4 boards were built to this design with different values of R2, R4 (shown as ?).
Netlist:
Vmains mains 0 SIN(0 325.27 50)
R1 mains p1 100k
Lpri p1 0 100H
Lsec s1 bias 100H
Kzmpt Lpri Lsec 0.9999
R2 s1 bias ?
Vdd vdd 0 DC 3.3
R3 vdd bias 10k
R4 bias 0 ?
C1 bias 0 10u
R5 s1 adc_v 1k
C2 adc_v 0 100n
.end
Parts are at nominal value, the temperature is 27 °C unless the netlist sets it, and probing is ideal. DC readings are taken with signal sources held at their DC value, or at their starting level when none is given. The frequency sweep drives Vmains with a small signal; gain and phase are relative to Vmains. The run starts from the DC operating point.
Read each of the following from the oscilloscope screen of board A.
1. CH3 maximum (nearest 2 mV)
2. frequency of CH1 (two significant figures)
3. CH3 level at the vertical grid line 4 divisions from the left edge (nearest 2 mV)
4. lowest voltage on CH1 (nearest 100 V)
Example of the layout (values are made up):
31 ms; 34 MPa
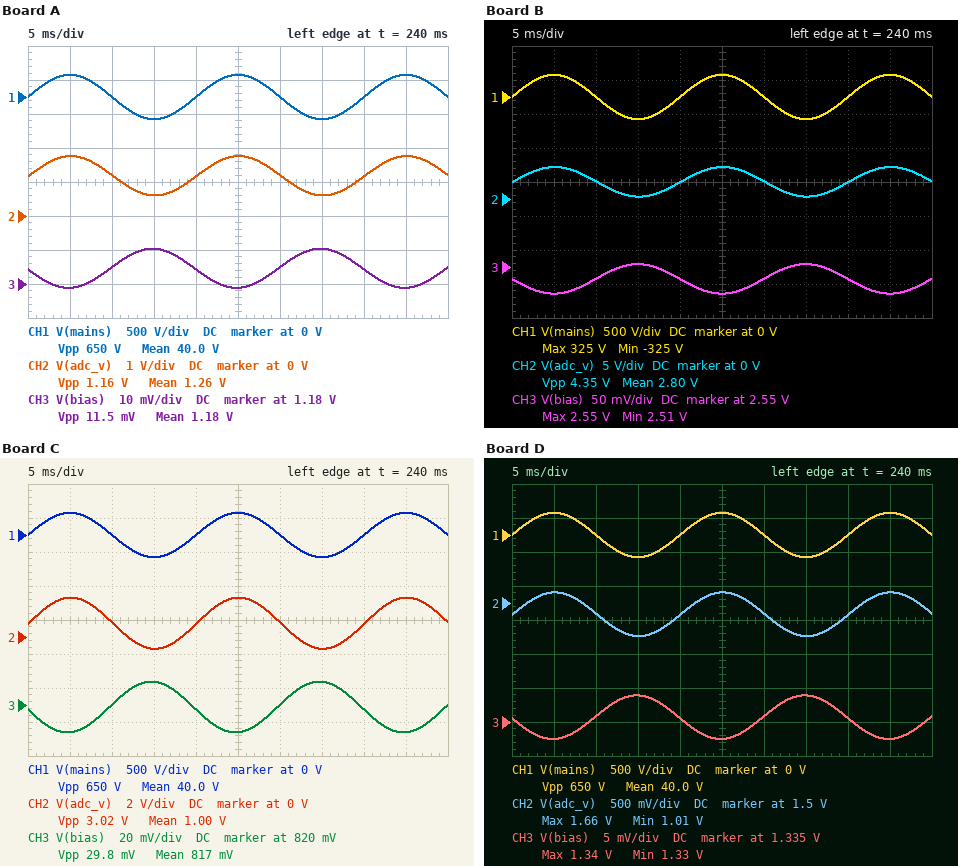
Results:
1.190 V; 50 Hz; 1.184 V; -300 V
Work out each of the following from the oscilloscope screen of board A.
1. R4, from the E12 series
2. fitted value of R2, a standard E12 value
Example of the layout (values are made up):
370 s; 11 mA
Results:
5.6 kΩ; 180 Ω
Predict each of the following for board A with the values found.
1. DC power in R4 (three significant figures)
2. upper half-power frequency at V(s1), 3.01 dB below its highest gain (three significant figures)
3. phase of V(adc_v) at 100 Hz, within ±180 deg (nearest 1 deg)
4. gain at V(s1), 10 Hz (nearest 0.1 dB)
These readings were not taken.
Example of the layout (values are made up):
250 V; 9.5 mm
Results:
251 µW; 539 kHz; -4 deg; -55.0 dB
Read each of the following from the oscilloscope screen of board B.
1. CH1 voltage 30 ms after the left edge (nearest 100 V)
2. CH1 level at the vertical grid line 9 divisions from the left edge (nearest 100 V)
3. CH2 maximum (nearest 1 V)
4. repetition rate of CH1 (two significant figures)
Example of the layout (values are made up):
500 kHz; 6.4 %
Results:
0 V; 300 V; 5 V; 50 Hz
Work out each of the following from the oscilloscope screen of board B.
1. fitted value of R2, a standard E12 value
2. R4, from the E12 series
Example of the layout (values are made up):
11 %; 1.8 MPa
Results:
680 Ω; 33 kΩ
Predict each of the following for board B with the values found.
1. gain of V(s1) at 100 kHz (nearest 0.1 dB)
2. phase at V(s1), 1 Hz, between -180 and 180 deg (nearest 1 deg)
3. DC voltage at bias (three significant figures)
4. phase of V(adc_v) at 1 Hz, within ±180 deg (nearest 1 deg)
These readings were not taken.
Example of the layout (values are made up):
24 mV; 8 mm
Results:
-48.0 dB; 47 deg; 2.53 V; 47 deg
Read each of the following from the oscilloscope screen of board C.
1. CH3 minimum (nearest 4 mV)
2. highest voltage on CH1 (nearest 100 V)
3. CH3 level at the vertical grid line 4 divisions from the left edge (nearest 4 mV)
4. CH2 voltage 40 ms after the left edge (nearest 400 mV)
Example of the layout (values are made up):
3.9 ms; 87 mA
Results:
804 mV; 300 V; 816 mV; 800 mV
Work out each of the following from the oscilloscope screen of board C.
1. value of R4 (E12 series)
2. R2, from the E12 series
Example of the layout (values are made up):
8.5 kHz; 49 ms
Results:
3.3 kΩ; 470 Ω
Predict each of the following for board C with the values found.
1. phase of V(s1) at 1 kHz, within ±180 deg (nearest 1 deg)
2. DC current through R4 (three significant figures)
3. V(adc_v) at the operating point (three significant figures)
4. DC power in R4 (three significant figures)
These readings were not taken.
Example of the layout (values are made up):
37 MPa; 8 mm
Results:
-10 deg; 248 µA; 819 mV; 203 µW
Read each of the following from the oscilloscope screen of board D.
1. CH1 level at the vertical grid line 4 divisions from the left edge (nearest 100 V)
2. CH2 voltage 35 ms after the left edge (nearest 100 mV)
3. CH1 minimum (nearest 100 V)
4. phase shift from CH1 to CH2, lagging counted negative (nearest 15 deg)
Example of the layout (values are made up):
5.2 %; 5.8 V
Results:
0 V; 1.0 V; -300 V; 0 deg
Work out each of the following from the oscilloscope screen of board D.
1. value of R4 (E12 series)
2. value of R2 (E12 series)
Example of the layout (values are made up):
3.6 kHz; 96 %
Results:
6.8 kΩ; 100 Ω
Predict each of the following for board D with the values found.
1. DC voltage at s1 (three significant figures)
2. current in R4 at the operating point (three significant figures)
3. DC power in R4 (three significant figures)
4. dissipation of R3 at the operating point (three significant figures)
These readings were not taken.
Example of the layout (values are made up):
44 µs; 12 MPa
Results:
1.34 V; 196 µA; 262 µW; 386 µW
